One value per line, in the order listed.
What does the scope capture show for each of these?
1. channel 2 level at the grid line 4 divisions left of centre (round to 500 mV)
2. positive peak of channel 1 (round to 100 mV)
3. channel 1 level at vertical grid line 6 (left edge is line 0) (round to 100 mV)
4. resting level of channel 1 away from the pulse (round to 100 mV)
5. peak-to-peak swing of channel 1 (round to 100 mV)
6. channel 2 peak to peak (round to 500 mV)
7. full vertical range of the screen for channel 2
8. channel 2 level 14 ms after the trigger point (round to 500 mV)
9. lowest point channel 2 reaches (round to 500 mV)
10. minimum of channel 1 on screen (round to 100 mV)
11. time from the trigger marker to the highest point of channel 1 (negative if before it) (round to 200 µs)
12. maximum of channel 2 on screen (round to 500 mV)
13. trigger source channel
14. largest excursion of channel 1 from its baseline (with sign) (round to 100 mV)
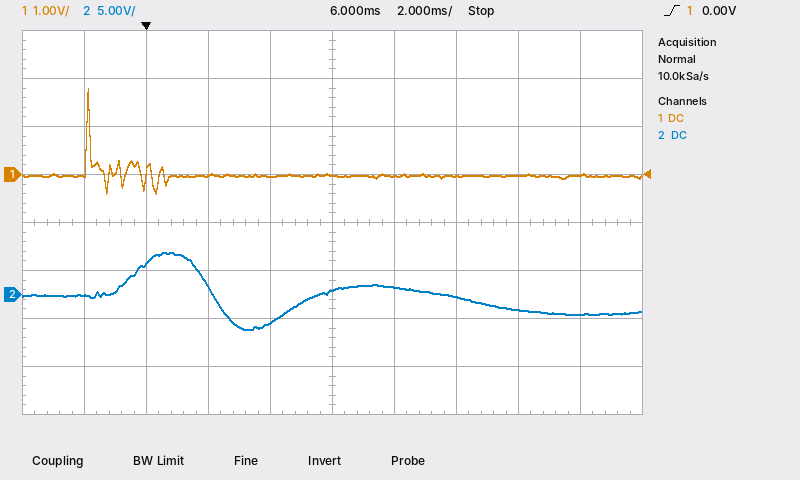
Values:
0.0 V
1.8 V
0.0 V
0.0 V
2.2 V
8.0 V
40 V
-2.0 V
-3.5 V
-400 mV
-1.8 ms
4.5 V
channel 1
+1.8 V
